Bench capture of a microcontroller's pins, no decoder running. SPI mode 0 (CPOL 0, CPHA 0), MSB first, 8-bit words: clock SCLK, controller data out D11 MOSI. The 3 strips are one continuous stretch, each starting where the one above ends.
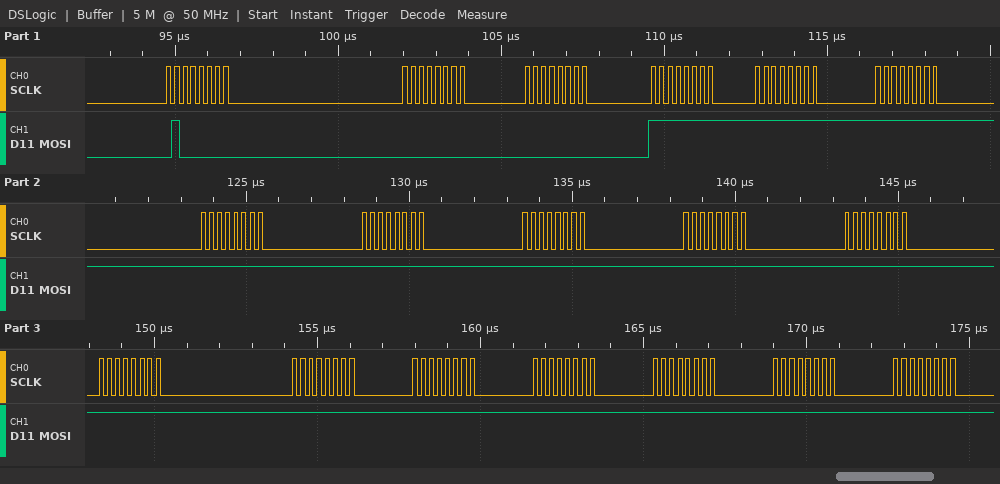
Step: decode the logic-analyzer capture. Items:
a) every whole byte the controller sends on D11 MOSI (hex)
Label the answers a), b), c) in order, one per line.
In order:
a) 40 00 00 FF FF FF FF FF FF FF FF FF FF FF FF FF FF FF
